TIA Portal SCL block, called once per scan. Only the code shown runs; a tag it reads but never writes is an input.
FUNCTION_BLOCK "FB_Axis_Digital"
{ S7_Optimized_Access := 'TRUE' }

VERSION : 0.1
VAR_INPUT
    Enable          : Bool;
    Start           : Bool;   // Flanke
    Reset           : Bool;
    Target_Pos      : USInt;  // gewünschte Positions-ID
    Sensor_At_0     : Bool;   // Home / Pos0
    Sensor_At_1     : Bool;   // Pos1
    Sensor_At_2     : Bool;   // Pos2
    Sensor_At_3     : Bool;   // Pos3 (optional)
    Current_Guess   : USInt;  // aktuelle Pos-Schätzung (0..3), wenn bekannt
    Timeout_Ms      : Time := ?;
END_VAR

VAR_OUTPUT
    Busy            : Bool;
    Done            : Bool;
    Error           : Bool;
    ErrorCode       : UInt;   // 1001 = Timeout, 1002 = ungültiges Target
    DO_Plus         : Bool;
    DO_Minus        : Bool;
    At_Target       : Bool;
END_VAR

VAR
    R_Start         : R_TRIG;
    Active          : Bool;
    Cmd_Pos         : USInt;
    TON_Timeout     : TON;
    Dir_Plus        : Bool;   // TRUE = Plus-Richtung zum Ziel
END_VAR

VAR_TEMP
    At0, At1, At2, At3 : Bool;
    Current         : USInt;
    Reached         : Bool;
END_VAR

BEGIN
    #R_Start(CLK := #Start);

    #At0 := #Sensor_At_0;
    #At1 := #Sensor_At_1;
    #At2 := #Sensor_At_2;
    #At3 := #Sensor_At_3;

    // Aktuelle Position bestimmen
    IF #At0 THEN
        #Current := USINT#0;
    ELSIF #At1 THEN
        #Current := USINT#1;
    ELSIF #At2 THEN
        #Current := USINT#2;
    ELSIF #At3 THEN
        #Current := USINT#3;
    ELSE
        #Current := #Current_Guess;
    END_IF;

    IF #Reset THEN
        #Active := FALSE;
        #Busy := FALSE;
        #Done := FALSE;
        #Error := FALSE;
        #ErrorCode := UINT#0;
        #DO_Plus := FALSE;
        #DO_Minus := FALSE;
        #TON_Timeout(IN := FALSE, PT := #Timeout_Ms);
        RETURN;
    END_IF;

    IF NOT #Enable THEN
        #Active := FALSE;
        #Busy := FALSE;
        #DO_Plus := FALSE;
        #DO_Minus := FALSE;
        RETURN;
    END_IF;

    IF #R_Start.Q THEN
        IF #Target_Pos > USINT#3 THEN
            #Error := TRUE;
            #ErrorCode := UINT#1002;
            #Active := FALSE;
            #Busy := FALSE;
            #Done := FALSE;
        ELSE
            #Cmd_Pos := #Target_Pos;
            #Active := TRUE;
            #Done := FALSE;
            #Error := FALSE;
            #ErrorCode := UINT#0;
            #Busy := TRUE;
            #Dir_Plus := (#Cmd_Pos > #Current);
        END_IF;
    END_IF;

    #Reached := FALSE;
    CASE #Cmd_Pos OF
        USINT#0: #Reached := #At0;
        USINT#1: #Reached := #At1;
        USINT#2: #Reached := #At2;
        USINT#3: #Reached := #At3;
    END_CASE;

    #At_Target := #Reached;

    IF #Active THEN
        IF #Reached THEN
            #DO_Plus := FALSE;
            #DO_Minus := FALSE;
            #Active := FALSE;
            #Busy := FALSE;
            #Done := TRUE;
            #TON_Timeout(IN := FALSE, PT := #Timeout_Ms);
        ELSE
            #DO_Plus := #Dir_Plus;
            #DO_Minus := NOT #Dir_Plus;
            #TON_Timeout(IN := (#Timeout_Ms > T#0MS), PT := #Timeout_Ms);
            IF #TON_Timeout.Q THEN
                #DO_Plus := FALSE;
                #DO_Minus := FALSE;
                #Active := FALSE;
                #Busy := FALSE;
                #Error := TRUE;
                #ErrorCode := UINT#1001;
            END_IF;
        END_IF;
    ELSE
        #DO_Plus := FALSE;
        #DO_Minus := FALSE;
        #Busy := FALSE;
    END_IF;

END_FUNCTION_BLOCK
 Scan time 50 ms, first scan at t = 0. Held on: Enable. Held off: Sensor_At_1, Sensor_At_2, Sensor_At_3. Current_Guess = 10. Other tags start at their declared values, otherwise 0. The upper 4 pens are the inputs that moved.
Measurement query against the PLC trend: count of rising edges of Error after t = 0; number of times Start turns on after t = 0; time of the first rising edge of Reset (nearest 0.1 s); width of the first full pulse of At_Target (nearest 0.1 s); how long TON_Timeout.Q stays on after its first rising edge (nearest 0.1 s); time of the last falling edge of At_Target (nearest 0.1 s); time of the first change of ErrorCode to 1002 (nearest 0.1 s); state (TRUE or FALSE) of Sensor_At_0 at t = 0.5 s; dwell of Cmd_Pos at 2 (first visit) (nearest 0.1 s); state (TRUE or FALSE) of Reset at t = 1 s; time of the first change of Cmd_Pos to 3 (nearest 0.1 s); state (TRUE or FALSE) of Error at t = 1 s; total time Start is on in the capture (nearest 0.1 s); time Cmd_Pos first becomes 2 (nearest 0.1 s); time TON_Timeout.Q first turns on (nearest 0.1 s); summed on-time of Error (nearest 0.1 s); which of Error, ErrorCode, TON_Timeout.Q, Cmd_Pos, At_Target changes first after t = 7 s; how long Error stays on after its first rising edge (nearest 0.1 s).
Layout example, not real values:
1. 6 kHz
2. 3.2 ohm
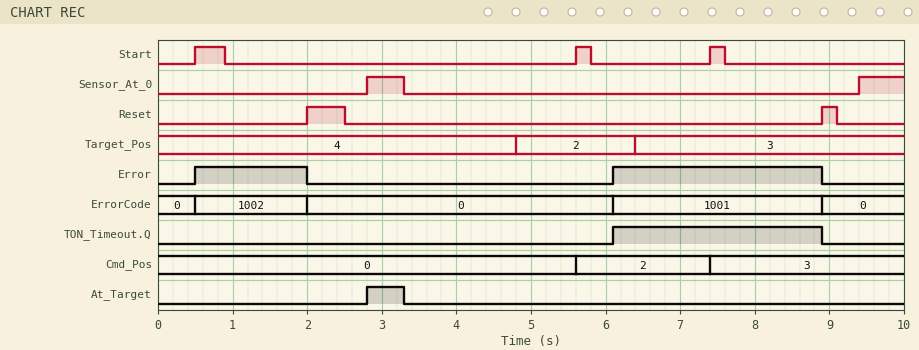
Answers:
1. 2
2. 3
3. 2.0 s
4. 0.5 s
5. 2.8 s
6. 3.3 s
7. 0.5 s
8. FALSE
9. 1.8 s
10. FALSE
11. 7.4 s
12. TRUE
13. 0.8 s
14. 5.6 s
15. 6.1 s
16. 4.3 s
17. Cmd_Pos
18. 1.5 s
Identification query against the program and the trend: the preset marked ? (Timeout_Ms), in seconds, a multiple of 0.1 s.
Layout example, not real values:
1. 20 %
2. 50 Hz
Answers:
1. 0.5 s
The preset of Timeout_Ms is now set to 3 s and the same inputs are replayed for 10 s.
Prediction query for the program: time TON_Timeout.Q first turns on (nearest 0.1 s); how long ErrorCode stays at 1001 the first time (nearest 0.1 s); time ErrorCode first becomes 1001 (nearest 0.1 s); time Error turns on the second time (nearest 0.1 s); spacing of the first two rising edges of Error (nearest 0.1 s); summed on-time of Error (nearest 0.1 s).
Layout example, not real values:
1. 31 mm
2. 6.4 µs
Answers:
1. 8.6 s
2. 0.3 s
3. 8.6 s
4. 8.6 s
5. 8.1 s
6. 1.8 s
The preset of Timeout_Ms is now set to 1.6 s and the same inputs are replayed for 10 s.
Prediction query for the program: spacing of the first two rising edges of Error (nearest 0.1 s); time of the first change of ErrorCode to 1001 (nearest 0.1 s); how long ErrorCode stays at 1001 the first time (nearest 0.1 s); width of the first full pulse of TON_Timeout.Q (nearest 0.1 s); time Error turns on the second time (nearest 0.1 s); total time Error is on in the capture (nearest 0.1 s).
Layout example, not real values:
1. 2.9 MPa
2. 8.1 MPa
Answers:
1. 6.7 s
2. 7.2 s
3. 1.7 s
4. 1.7 s
5. 7.2 s
6. 3.2 s
